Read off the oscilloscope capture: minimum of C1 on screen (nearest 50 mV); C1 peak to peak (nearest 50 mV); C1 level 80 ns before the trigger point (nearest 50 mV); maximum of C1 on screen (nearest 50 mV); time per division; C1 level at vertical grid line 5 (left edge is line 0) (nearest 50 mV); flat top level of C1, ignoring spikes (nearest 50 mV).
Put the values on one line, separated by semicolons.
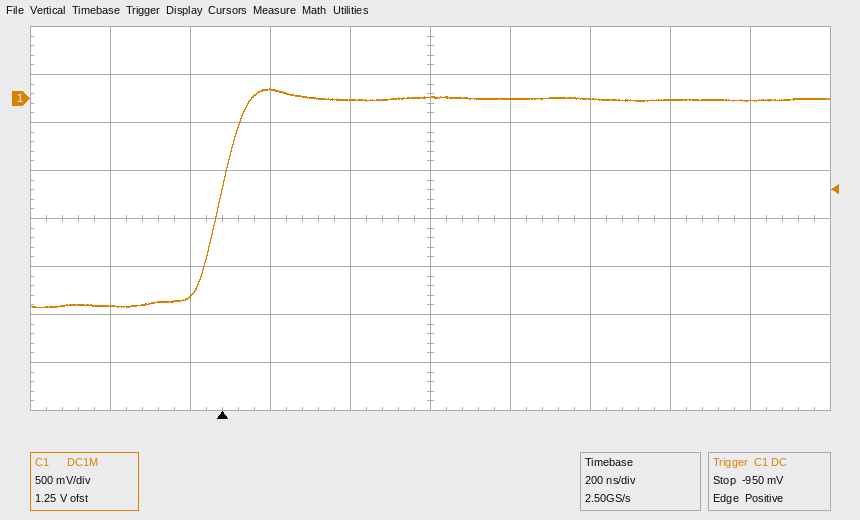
-2.20 V; 2.30 V; -2.05 V; 100 mV; 200 ns; 0 mV; 0 mV
